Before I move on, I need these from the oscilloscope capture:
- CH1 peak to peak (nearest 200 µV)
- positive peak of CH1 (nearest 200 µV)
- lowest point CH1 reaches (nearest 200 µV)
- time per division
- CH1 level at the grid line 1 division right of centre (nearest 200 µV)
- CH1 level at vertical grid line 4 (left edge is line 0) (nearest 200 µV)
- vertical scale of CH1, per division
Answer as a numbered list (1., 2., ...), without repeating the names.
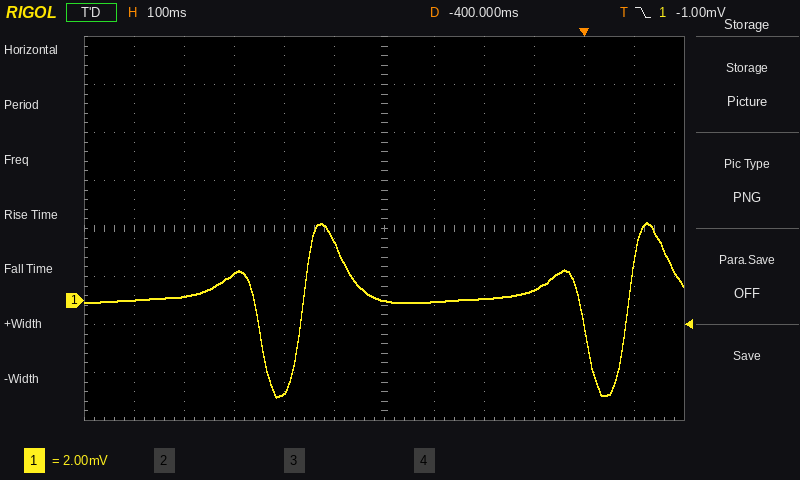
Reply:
1. 7.2 mV
2. 3.2 mV
3. -4.0 mV
4. 100 ms
5. 0.0 mV
6. -3.8 mV
7. 2 mV
